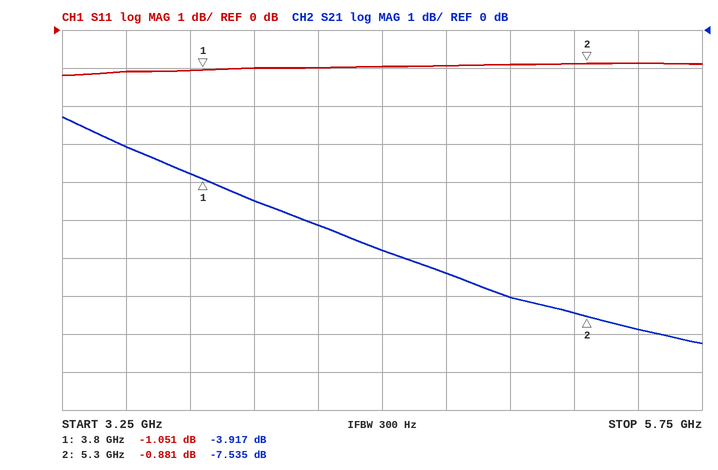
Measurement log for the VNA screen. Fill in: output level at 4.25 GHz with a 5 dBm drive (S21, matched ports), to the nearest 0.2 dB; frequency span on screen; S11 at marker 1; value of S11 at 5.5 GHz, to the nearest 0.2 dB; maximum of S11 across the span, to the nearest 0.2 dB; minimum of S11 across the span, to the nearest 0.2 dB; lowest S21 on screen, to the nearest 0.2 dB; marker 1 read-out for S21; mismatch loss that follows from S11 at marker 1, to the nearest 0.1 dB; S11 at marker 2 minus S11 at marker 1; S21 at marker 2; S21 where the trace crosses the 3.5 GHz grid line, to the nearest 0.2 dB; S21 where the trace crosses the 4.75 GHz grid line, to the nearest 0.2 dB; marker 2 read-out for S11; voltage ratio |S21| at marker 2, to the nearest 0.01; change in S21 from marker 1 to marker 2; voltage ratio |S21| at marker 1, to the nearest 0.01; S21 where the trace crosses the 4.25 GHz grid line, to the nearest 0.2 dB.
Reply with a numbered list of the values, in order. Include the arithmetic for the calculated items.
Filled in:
1. 5 dBm + (-5.2 dB) = -0.2 dBm
2. 2.5 GHz
3. -1.051 dB
4. -0.8 dB
5. -0.8 dB
6. -1.2 dB
7. -8.2 dB
8. -3.917 dB
9. −10 log10(1 − 10^(-1.051/10)) ≈ 6.7 dB
10. -0.881 − (-1.051) = 0.170 dB
11. -7.535 dB
12. -3.0 dB
13. -6.4 dB
14. -0.881 dB
15. 10^(-7.535/20) ≈ 0.42
16. -7.535 − (-3.917) = -3.618 dB
17. 10^(-3.917/20) ≈ 0.64
18. -5.2 dB
